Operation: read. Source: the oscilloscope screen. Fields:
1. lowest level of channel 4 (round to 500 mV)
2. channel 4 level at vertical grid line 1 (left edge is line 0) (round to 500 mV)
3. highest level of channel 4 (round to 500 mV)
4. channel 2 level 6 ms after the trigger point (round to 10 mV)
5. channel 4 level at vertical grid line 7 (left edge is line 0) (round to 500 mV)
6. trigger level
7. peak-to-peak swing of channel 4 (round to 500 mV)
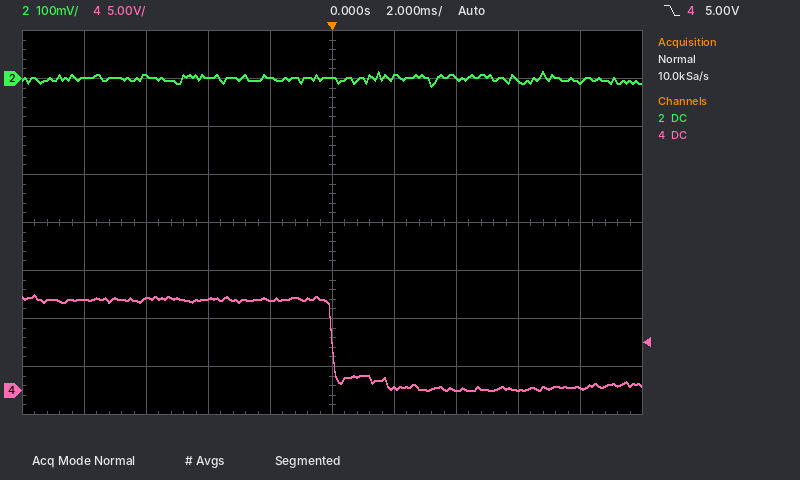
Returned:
0.0 V
9.5 V
10.0 V
0 mV
0.0 V
5.00 V
10.0 V
